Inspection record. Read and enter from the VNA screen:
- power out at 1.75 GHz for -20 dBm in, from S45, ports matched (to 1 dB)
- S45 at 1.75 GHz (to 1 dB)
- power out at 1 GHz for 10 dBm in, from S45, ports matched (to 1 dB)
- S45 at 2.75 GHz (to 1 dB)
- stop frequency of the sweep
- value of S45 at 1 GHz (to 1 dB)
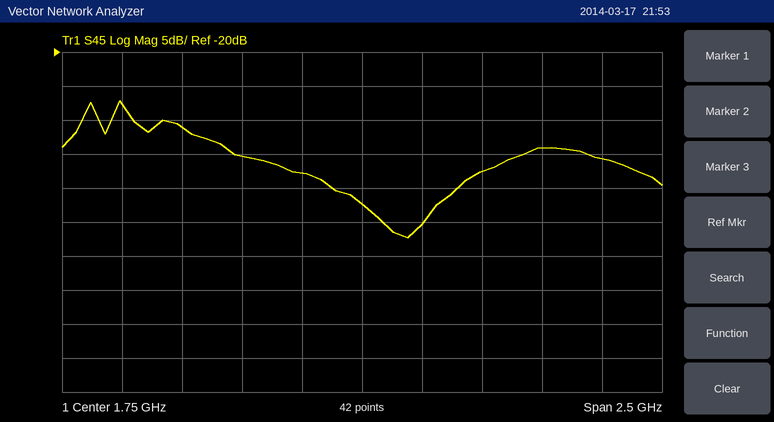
-62 dBm
-42 dB
-21 dBm
-36 dB
3 GHz
-31 dB
